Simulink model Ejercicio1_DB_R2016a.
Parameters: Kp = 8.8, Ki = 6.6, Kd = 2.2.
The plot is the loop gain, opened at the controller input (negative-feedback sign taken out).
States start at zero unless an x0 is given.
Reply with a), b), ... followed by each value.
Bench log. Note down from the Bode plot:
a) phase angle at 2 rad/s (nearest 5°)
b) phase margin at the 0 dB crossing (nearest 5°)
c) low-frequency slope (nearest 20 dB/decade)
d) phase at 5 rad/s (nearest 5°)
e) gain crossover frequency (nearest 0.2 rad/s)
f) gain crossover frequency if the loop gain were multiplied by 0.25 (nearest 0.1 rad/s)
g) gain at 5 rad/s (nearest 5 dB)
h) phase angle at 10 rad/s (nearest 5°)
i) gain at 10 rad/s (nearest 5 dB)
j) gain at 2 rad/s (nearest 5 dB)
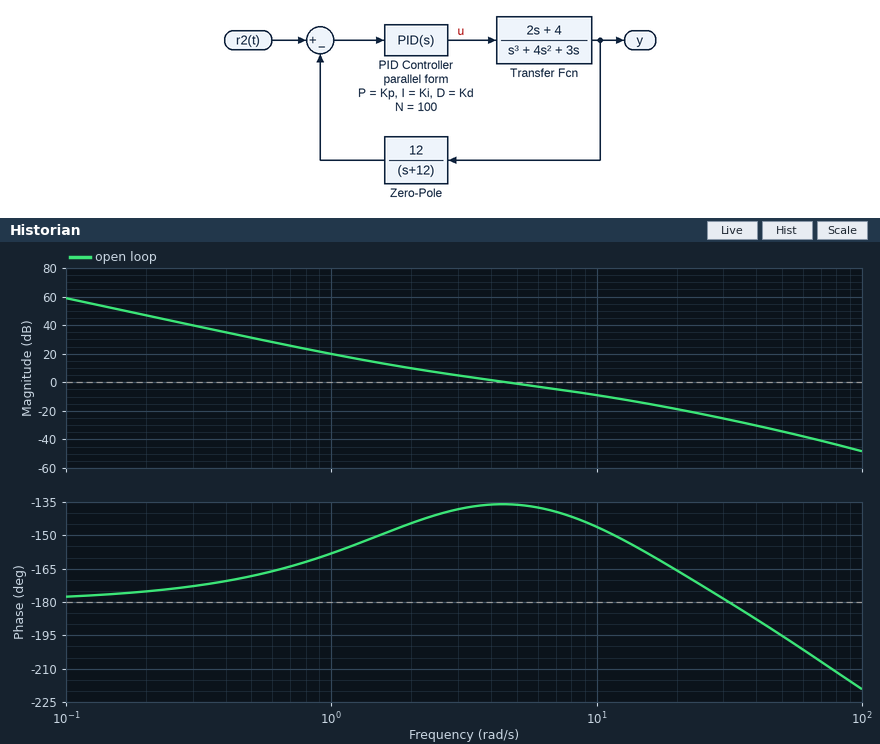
a) -145°
b) 45°
c) -40 dB/decade
d) -135°
e) 4.6 rad/s
f) 1.7 rad/s
g) 0 dB
h) -145°
i) -10 dB
j) 10 dB
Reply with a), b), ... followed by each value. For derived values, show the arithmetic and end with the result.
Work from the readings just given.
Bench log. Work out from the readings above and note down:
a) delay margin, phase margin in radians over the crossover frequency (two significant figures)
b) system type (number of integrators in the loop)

a) 45 × π / 180 / 4.6 = 0.17 s
b) 2
